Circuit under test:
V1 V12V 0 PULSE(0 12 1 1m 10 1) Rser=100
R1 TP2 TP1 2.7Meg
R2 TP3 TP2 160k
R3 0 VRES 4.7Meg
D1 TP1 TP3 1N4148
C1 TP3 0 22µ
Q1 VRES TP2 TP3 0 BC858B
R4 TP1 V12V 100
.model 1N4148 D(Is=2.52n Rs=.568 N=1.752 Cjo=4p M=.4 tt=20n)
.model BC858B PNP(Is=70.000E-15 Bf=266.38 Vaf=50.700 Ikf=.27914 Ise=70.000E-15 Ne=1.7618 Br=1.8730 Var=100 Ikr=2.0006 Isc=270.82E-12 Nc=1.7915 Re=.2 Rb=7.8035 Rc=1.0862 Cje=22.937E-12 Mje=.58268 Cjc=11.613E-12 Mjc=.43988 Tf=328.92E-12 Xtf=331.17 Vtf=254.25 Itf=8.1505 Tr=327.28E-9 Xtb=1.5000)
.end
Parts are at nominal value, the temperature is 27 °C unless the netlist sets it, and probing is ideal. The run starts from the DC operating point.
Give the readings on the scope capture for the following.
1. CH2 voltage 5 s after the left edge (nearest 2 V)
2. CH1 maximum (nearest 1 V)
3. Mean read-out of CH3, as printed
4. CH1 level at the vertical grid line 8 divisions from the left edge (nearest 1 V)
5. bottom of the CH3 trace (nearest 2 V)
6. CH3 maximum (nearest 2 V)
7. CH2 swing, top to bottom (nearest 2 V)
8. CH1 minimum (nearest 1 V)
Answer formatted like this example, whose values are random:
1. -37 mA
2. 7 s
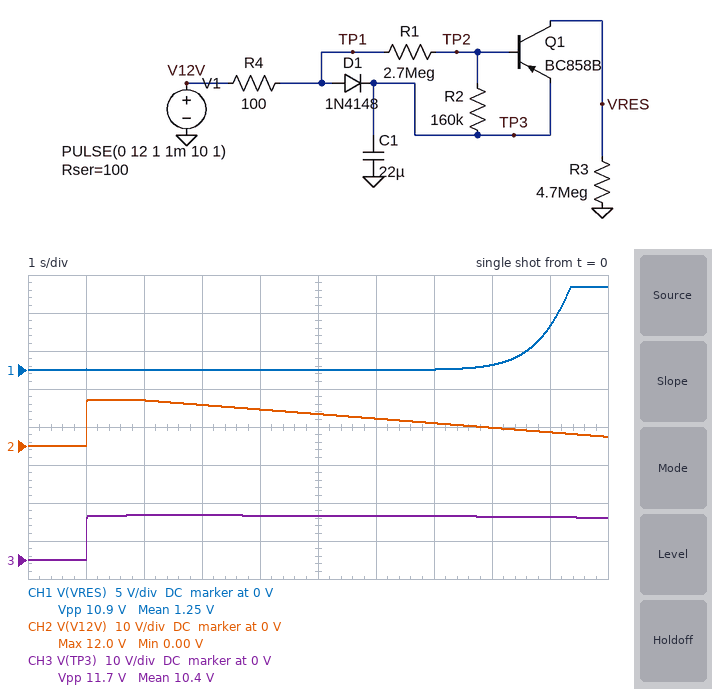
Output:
1. 8 V
2. 11 V
3. 10.4 V
4. 1 V
5. 0 V
6. 12 V
7. 12 V
8. 0 V
